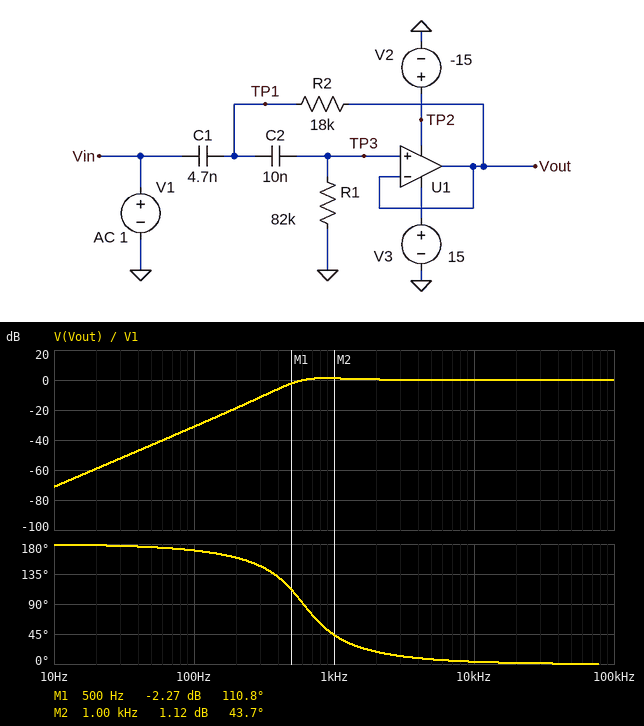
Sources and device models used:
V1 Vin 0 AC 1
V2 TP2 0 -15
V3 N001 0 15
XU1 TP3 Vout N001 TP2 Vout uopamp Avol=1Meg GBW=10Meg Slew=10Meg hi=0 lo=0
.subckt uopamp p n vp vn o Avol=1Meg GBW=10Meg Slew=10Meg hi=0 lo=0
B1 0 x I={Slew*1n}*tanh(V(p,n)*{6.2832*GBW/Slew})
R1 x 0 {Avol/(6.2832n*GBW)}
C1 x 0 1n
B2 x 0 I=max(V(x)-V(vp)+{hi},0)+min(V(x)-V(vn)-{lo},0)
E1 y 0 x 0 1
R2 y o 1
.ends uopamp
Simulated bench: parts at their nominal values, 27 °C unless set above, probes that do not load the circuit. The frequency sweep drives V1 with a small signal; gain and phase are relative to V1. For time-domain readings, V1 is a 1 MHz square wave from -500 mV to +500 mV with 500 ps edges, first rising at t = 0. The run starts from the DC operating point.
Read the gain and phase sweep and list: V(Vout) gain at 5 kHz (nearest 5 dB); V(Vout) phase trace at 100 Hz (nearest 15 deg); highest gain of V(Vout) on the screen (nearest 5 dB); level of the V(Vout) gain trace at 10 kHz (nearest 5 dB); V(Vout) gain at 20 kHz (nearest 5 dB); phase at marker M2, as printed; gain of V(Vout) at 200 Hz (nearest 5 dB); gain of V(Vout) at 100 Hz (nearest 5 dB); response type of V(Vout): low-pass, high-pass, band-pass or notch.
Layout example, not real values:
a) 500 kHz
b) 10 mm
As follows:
a) 0 dB
b) 165 deg
c) 0 dB
d) 0 dB
e) 0 dB
f) 43.7 deg
g) -20 dB
h) -30 dB
i) high-pass
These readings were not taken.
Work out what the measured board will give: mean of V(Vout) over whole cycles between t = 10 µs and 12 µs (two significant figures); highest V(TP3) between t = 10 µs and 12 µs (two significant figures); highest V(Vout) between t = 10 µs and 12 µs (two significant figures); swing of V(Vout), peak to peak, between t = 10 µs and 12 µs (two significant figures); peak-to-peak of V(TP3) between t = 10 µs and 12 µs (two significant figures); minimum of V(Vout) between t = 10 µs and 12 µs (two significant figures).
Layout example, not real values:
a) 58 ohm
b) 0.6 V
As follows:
a) 480 mV
b) 980 mV
c) 980 mV
d) 1.0 V
e) 1.0 V
f) -23 mV
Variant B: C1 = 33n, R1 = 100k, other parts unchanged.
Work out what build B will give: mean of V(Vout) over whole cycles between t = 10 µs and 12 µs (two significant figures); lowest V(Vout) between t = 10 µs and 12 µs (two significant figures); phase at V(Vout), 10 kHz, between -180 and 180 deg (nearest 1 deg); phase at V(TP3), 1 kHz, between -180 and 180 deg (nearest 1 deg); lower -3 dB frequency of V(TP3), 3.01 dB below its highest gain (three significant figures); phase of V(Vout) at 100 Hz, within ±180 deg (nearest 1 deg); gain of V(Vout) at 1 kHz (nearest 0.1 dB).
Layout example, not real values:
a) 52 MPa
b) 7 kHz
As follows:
a) 490 mV
b) -7.8 mV
c) 1 deg
d) 12 deg
e) 177 Hz
f) 148 deg
g) 0.2 dB
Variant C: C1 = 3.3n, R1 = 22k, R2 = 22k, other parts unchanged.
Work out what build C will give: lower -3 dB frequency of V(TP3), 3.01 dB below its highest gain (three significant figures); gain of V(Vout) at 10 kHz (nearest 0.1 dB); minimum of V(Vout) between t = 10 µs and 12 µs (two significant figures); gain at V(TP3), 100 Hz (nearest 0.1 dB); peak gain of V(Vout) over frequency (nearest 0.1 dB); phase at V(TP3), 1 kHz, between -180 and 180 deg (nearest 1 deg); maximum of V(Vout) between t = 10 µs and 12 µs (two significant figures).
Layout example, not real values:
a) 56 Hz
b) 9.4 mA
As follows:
a) 2.40 kHz
b) -0.2 dB
c) -100 mV
d) -44.1 dB
e) 0 dB
f) 101 deg
g) 910 mV
